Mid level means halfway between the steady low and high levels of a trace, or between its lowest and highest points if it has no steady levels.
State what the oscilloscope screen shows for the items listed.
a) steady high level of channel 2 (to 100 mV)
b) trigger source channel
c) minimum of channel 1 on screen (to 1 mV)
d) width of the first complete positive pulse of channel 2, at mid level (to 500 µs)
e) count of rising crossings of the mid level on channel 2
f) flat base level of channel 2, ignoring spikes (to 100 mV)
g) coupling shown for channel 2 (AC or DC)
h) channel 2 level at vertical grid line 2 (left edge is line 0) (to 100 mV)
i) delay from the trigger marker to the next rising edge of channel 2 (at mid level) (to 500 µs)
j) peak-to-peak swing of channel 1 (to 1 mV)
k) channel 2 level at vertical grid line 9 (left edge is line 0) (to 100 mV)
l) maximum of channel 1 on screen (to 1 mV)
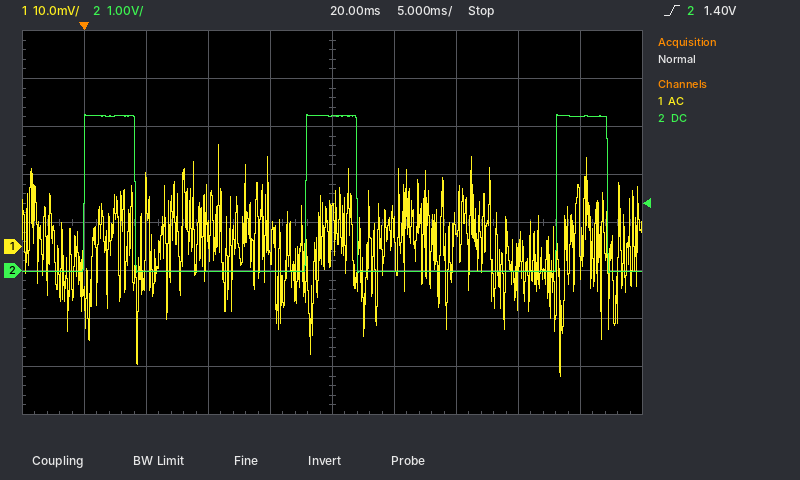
3.2 V
channel 2
-27 mV
4.0 ms
3
0.0 V
DC
0.0 V
18.0 ms
48 mV
3.2 V
21 mV
